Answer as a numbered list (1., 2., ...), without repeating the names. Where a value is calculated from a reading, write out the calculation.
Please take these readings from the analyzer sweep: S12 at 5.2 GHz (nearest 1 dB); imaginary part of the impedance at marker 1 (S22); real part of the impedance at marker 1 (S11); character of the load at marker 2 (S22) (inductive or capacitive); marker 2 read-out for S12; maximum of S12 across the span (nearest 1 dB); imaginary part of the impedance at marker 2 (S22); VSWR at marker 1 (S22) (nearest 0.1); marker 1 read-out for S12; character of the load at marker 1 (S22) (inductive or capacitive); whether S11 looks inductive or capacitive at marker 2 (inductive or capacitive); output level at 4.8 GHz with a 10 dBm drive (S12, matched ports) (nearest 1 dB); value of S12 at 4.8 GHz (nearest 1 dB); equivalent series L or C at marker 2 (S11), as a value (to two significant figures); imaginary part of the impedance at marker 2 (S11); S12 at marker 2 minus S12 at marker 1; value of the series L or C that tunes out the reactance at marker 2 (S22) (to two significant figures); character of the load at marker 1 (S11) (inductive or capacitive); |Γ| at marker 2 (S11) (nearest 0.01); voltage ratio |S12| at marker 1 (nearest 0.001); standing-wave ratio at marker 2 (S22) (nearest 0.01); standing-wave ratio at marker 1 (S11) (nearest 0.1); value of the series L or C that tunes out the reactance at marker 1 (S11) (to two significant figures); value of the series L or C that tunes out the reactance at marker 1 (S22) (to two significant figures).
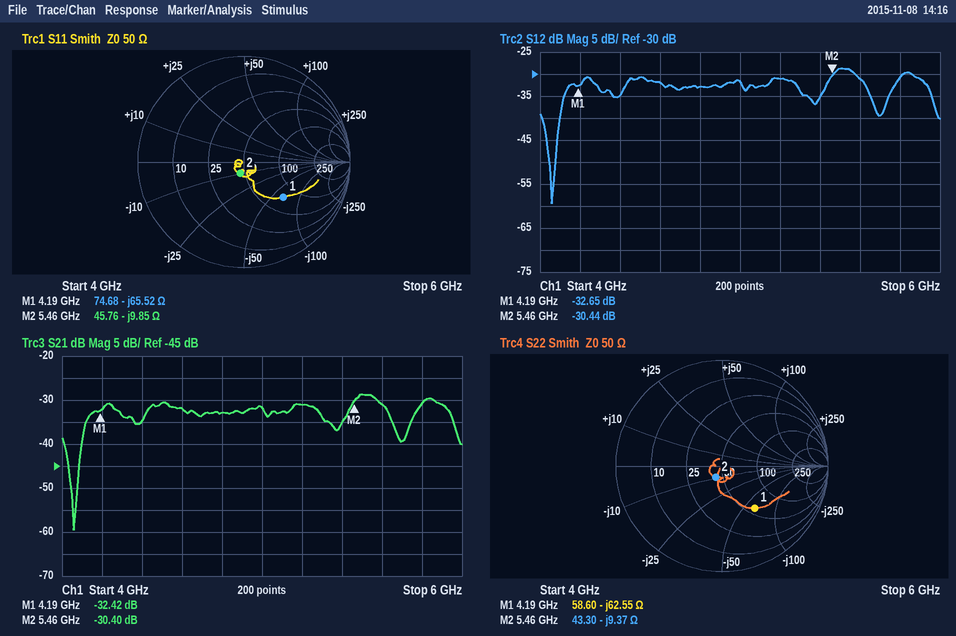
1. -31 dB
2. -62.55 Ω
3. 74.68 Ω
4. capacitive
5. -30.44 dB
6. -29 dB
7. -9.37 Ω
8. 3.0
9. -32.65 dB
10. capacitive
11. capacitive
12. 10 dBm + (-33 dB) = -23 dBm
13. -33 dB
14. C = 1/(2π × 5.46 GHz × 9.85 Ω) ≈ 3.0 pF
15. -9.85 Ω
16. -30.44 − (-32.65) = 2.21 dB
17. L = 9.37 Ω/(2π × 5.46 GHz) ≈ 273 pH, so 270 pH to two significant figures
18. capacitive
19. 0.11
20. 10^(-32.65/20) ≈ 0.023
21. 1.28
22. 3.0
23. L = 65.52 Ω/(2π × 4.19 GHz) ≈ 2.5 nH
24. L = 62.55 Ω/(2π × 4.19 GHz) ≈ 2.4 nH
